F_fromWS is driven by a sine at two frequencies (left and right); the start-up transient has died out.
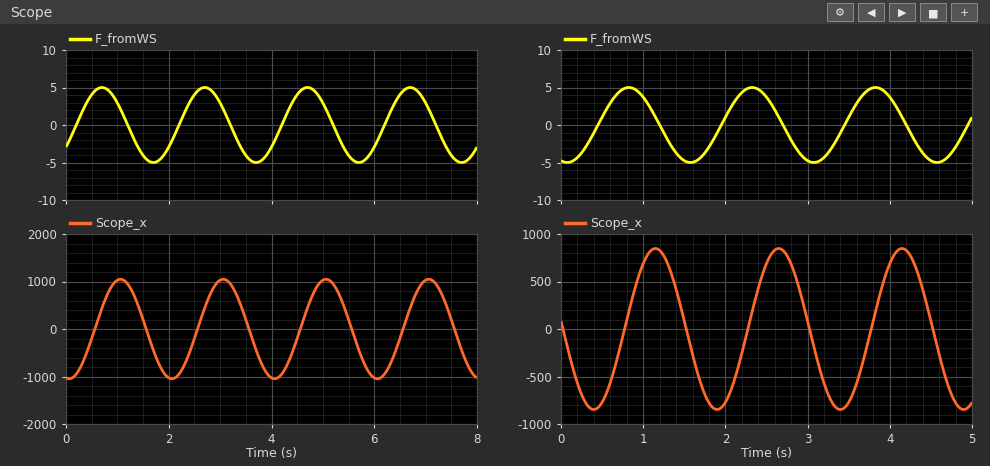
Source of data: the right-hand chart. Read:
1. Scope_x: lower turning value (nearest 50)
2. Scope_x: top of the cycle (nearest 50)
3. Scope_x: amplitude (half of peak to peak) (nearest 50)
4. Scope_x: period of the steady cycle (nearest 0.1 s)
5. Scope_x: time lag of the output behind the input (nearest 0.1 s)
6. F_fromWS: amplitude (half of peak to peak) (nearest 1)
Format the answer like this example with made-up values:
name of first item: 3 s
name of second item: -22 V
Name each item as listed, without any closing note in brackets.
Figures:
Scope_x: lower turning value: -850
Scope_x: top of the cycle: 850
Scope_x: amplitude (half of peak to peak): 850
Scope_x: period of the steady cycle: 1.5 s
Scope_x: time lag of the output behind the input: 0.3 s
F_fromWS: amplitude (half of peak to peak): 5
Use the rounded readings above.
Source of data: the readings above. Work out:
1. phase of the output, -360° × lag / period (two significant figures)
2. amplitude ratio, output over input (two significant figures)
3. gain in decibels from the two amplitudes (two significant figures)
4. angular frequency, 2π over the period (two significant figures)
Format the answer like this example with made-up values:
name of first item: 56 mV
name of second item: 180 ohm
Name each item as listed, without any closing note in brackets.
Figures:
phase of the output, -360° × lag / period: -72°
amplitude ratio, output over input: 170
gain in decibels from the two amplitudes: 45 dB
angular frequency, 2π over the period: 4.2 rad/s
